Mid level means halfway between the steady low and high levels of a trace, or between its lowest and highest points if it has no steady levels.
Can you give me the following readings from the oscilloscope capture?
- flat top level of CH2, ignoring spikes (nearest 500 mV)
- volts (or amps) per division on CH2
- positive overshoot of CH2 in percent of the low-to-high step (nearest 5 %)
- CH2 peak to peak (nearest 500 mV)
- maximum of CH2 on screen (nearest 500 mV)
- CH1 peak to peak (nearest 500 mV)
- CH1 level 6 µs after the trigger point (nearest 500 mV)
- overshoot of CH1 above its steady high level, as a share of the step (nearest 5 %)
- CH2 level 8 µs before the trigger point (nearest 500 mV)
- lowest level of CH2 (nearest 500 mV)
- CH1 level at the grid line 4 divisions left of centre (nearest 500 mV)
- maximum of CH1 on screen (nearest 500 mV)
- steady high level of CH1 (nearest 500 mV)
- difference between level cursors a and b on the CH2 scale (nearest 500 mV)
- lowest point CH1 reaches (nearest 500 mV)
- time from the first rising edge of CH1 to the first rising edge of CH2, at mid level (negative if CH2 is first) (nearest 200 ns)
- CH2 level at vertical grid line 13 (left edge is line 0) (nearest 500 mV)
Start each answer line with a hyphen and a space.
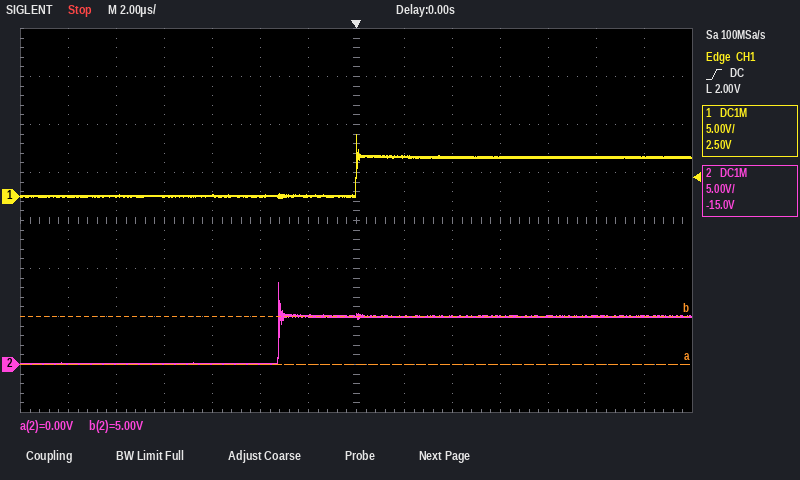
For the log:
- 5.0 V
- 5 V
- 70 %
- 8.5 V
- 8.5 V
- 6.5 V
- 4.0 V
- 60 %
- 0.0 V
- 0.0 V
- 0.0 V
- 6.5 V
- 4.0 V
- 5.0 V
- 0.0 V
- -3.2 µs
- 5.0 V
